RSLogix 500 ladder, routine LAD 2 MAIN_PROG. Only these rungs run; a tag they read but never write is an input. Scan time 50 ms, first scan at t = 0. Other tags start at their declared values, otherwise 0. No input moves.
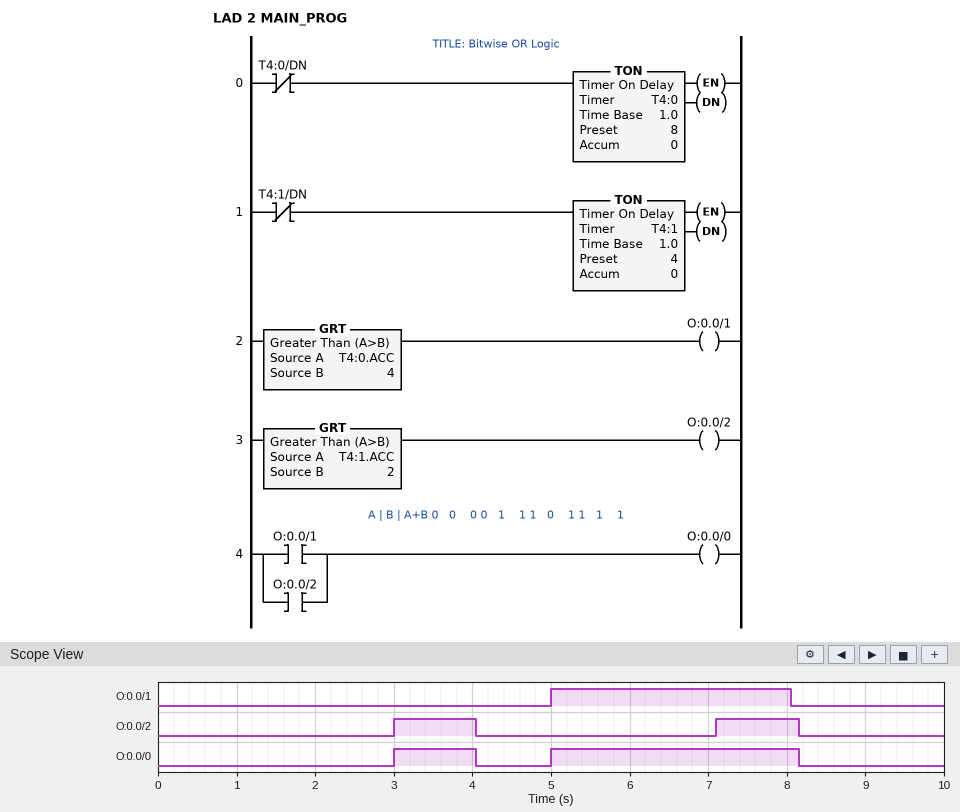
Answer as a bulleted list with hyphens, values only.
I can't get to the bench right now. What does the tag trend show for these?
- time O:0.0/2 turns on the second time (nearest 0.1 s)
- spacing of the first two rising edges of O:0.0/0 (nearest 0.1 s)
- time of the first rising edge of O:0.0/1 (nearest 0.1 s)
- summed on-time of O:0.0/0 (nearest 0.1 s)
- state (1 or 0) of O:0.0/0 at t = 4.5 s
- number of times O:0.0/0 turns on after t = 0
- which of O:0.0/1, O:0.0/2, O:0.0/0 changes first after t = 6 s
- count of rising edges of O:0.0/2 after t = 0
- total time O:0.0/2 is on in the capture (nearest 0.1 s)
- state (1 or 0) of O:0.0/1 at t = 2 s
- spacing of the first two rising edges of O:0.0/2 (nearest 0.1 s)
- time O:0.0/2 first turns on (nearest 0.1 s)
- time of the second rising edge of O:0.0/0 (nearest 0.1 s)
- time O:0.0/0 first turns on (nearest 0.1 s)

- 7.1 s
- 2.0 s
- 5.0 s
- 4.2 s
- 0
- 2
- O:0.0/2
- 2
- 2.1 s
- 0
- 4.1 s
- 3.0 s
- 5.0 s
- 3.0 s
